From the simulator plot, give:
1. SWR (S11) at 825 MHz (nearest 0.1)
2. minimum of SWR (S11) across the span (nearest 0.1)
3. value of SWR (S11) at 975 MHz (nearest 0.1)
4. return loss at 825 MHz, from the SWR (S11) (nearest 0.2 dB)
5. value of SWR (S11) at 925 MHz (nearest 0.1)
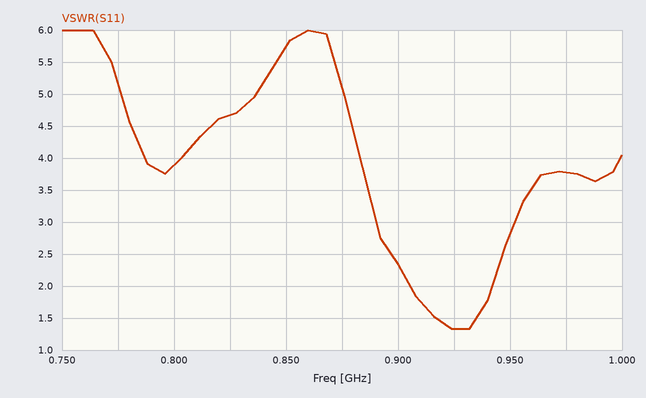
4.7
1.3
3.8
3.8 dB
1.3
